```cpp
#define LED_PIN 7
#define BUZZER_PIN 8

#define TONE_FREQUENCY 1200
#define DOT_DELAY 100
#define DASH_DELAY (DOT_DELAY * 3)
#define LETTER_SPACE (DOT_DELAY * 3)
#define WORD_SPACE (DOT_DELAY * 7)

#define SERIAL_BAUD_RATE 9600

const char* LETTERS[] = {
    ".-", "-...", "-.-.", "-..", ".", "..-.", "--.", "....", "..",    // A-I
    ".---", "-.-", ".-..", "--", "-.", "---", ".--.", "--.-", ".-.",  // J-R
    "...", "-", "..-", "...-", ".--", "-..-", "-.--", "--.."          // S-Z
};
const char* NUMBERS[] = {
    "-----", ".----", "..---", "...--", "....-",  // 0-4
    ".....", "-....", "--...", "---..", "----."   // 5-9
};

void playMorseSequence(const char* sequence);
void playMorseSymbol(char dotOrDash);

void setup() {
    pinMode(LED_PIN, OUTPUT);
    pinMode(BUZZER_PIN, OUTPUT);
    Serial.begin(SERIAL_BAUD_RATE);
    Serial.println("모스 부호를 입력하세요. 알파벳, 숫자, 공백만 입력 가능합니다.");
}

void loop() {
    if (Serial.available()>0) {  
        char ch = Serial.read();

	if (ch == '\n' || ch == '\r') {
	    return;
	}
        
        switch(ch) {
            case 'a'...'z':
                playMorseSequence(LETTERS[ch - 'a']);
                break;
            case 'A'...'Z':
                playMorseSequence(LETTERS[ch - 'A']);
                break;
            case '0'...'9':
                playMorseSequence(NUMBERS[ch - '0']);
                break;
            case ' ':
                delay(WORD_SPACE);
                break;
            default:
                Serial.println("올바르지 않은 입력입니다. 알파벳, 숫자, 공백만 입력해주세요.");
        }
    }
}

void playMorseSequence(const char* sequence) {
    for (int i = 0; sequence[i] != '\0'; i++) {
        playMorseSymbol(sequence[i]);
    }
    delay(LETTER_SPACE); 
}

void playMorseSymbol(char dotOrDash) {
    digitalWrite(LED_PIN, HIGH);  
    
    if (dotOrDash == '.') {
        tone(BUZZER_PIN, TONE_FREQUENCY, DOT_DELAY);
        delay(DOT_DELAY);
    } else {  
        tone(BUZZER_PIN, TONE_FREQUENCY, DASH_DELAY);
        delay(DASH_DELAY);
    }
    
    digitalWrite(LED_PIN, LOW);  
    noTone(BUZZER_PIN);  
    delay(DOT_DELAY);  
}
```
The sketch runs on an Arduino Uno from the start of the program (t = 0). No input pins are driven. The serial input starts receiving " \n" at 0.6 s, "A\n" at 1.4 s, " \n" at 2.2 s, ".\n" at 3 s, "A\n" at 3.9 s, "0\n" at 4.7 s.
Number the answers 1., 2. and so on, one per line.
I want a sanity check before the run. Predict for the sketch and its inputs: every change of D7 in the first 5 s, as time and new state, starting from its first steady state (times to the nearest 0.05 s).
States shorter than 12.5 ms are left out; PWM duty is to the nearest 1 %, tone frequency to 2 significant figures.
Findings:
1. 0 s low; 1.4 s high; 1.5 s low; 1.6 s high; 1.9 s low; 3.9 s high; 4 s low; 4.1 s high; 4.4 s low; 4.8 s high
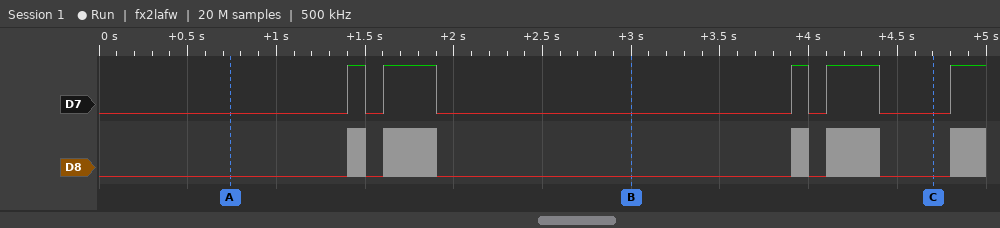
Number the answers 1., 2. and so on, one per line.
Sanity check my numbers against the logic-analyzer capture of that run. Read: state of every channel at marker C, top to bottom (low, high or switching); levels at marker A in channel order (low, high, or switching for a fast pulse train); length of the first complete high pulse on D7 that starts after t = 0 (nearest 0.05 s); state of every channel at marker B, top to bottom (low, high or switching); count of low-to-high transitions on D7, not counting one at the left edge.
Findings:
1. D7 low, D8 low
2. D7 low, D8 low
3. 0.10 s
4. D7 low, D8 low
5. 5
